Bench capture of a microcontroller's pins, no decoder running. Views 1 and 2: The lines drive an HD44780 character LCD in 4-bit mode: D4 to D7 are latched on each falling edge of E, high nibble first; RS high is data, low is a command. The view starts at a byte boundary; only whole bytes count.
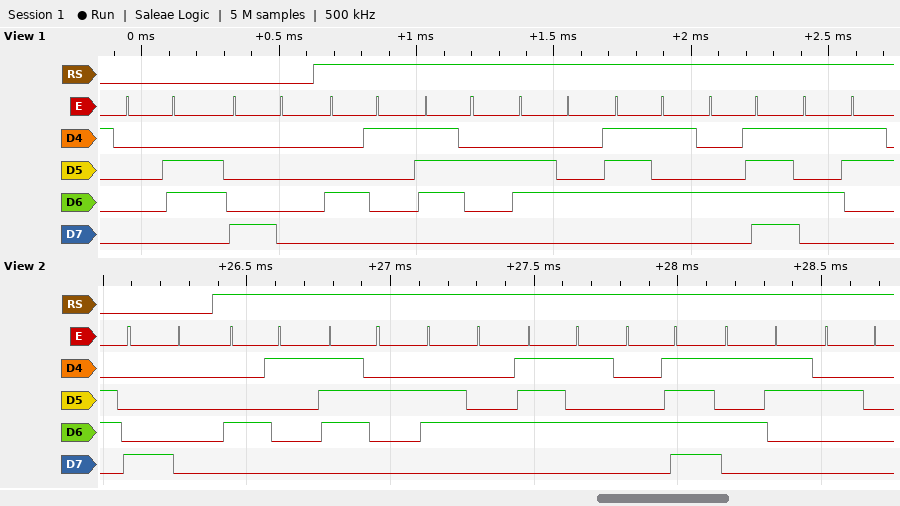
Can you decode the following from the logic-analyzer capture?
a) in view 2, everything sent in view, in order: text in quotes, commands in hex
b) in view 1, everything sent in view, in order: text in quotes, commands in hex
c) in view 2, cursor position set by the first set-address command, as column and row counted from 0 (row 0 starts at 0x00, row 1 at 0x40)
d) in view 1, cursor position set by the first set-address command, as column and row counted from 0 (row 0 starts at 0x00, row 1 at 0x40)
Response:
0x80 "ArduOS "
0x06 0x80 "ArduOS"
column 0, row 0
column 0, row 0
